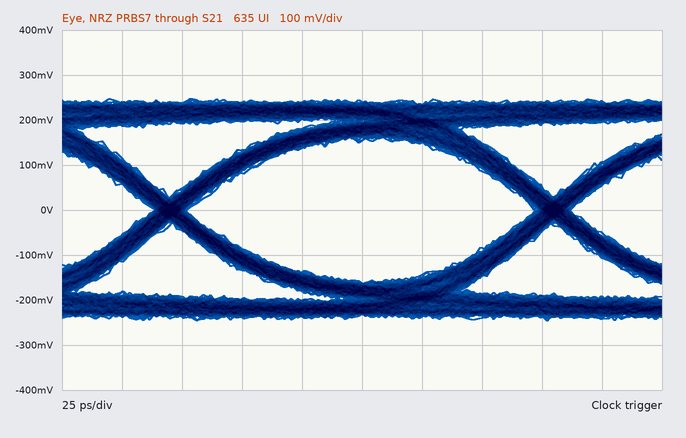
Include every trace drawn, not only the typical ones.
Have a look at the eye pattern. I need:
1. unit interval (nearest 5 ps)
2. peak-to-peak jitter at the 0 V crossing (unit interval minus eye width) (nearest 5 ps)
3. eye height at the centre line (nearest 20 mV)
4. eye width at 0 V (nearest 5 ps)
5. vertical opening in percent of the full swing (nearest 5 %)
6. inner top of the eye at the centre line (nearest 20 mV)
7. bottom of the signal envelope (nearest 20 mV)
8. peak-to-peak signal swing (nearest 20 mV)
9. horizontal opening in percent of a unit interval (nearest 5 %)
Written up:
160 ps
15 ps
320 mV
145 ps
65 %
160 mV
-240 mV
500 mV
90 %
